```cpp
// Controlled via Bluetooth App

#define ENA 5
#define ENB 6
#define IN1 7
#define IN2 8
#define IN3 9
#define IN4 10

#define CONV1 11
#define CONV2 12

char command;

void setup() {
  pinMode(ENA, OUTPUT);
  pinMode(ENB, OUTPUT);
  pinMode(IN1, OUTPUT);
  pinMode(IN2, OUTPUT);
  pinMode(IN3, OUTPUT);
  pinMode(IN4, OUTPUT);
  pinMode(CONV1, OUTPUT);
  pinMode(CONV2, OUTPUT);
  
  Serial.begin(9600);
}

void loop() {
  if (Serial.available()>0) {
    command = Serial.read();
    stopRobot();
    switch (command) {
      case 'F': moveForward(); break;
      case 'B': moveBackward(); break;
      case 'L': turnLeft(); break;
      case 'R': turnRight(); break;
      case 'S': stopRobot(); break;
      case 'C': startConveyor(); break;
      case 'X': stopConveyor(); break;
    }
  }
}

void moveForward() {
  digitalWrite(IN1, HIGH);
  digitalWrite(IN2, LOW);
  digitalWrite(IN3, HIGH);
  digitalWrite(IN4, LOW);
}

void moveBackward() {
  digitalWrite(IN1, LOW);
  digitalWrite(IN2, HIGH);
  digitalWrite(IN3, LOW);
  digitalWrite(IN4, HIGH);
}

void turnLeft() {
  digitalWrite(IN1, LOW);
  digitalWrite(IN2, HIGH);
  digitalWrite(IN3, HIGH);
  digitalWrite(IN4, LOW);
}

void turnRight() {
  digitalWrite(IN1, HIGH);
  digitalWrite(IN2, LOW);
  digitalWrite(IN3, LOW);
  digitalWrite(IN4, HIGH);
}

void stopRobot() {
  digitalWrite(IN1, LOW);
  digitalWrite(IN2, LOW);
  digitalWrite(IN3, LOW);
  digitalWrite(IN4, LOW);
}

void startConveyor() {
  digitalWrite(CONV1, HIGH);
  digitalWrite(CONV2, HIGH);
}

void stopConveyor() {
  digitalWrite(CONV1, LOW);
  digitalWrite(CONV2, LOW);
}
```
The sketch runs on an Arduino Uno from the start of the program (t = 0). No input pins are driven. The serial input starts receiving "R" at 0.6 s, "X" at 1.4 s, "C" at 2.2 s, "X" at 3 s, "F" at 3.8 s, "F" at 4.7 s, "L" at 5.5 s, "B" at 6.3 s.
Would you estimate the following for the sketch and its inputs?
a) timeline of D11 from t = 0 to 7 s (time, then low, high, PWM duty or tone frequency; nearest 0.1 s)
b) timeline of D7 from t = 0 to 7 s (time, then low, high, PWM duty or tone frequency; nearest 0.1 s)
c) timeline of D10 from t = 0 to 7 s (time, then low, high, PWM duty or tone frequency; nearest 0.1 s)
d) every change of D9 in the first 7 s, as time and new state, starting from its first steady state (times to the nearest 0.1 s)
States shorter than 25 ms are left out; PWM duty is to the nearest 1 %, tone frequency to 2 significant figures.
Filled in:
0 s low; 2.2 s high; 3 s low
0 s low; 0.6 s high; 1.4 s low; 3.8 s high; 5.5 s low
0 s low; 0.6 s high; 1.4 s low; 6.3 s high
0 s low; 3.8 s high; 6.3 s low
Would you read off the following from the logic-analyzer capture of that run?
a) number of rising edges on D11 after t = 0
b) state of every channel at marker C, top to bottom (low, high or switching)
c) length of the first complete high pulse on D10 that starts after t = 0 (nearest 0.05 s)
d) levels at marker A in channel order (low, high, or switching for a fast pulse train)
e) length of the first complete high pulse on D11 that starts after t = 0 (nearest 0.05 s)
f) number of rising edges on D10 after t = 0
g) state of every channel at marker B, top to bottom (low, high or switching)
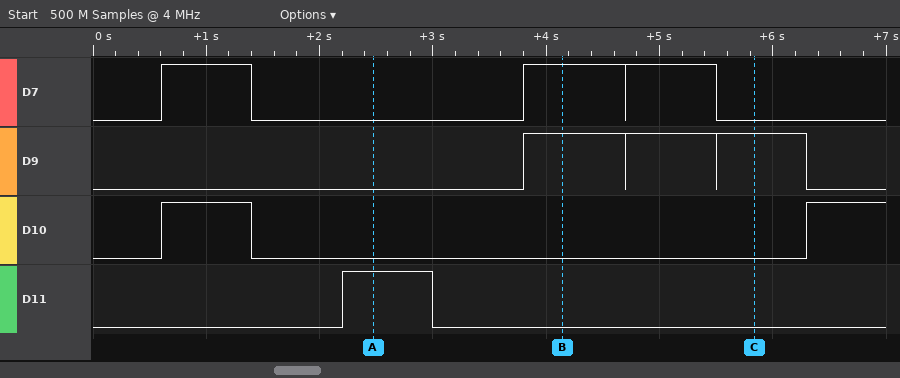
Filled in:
1
D7 low, D9 high, D10 low, D11 low
0.80 s
D7 low, D9 low, D10 low, D11 high
0.80 s
2
D7 high, D9 high, D10 low, D11 low
